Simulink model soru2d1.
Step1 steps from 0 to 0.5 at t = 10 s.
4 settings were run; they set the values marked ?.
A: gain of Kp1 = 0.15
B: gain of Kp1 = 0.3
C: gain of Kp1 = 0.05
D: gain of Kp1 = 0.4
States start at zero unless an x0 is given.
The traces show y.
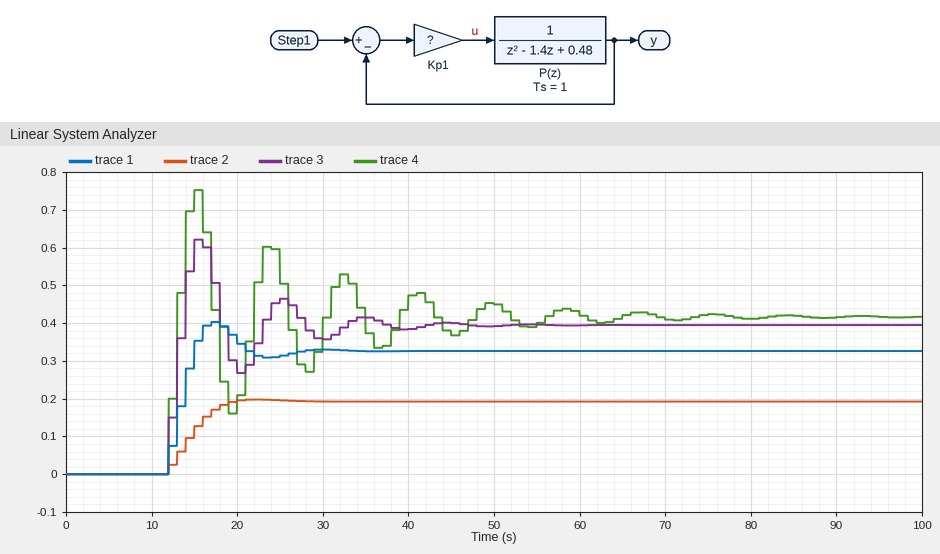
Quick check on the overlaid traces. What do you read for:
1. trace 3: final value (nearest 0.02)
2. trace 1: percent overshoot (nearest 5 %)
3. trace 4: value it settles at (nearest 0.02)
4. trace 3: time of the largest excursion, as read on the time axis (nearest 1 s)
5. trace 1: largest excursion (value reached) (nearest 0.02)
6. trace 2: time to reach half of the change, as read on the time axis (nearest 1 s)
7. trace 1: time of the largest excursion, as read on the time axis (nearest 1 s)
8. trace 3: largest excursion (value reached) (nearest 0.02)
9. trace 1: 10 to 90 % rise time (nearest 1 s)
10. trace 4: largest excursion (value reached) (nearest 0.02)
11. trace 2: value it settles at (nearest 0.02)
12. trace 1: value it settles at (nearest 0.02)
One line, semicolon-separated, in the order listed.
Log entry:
0.40; 25 %; 0.42; 15 s; 0.40; 15 s; 17 s; 0.62; 3 s; 0.76; 0.20; 0.32
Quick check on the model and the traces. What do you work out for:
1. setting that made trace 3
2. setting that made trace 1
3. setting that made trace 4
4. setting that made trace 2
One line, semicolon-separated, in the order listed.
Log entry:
B; A; D; C
